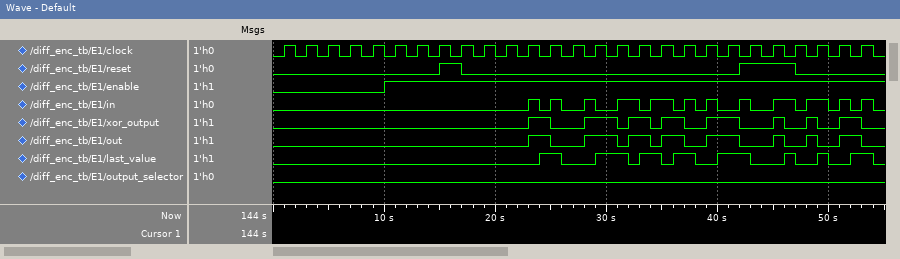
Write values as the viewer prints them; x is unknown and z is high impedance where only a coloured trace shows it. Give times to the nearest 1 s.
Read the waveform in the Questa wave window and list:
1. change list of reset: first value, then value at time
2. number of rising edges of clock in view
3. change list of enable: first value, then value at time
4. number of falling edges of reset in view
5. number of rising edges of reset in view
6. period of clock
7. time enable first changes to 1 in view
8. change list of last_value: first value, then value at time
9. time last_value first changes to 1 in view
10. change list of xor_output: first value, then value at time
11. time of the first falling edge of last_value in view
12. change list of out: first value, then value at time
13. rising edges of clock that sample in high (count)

0, 1 at 15 s, 0 at 17 s, 1 at 42 s, 0 at 47 s
27
0, 1 at 10 s
2
2
2 s
10 s
0, 1 at 24 s, 0 at 26 s, 1 at 29 s, 0 at 32 s, 1 at 33 s, 0 at 35 s, 1 at 36 s, 0 at 38 s, 1 at 40 s, 0 at 43 s, 1 at 46 s, 0 at 47 s, 1 at 49 s, 0 at 50 s, 1 at 52 s, 0 at 54 s
24 s
0, 1 at 23 s, 0 at 25 s, 1 at 28 s, 0 at 31 s, 1 at 32 s, 0 at 34 s, 1 at 35 s, 0 at 37 s, 1 at 39 s, 0 at 42 s, 1 at 45 s, 0 at 46 s, 1 at 48 s, 0 at 49 s, 1 at 51 s, 0 at 53 s
26 s
0, 1 at 23 s, 0 at 25 s, 1 at 28 s, 0 at 31 s, 1 at 32 s, 0 at 34 s, 1 at 35 s, 0 at 37 s, 1 at 39 s, 0 at 42 s, 1 at 45 s, 0 at 46 s, 1 at 48 s, 0 at 49 s, 1 at 51 s, 0 at 53 s
6
